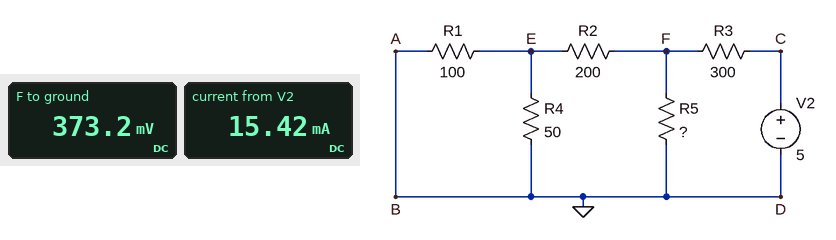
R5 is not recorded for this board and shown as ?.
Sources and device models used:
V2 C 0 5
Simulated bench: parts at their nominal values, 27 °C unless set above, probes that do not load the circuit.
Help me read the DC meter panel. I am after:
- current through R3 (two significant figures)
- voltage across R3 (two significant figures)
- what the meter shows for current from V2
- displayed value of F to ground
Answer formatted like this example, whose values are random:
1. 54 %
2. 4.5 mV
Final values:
1. 15 mA
2. 4.6 V
3. 15.42 mA
4. 373.2 mV
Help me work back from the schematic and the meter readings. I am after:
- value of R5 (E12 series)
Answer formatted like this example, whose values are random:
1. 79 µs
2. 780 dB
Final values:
1. 27 Ω
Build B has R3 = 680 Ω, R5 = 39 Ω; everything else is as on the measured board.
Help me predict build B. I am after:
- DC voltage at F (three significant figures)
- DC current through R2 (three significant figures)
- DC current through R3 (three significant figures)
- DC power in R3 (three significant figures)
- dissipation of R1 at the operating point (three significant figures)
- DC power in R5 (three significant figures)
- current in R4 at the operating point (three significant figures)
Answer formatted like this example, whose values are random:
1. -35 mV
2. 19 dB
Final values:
1. 234 mV
2. 1.00 mA
3. 7.01 mA
4. 33.4 mW
5. 11.2 µW
6. 1.41 mW
7. 669 µA
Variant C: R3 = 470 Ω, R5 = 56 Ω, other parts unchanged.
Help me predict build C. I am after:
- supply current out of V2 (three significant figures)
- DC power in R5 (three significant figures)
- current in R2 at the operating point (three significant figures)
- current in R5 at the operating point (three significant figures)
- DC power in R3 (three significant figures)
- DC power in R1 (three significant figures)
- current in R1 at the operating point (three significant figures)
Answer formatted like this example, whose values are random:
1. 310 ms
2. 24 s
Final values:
1. 9.71 mA
2. 3.43 mW
3. 1.88 mA
4. 7.83 mA
5. 44.3 mW
6. 39.2 µW
7. 626 µA
